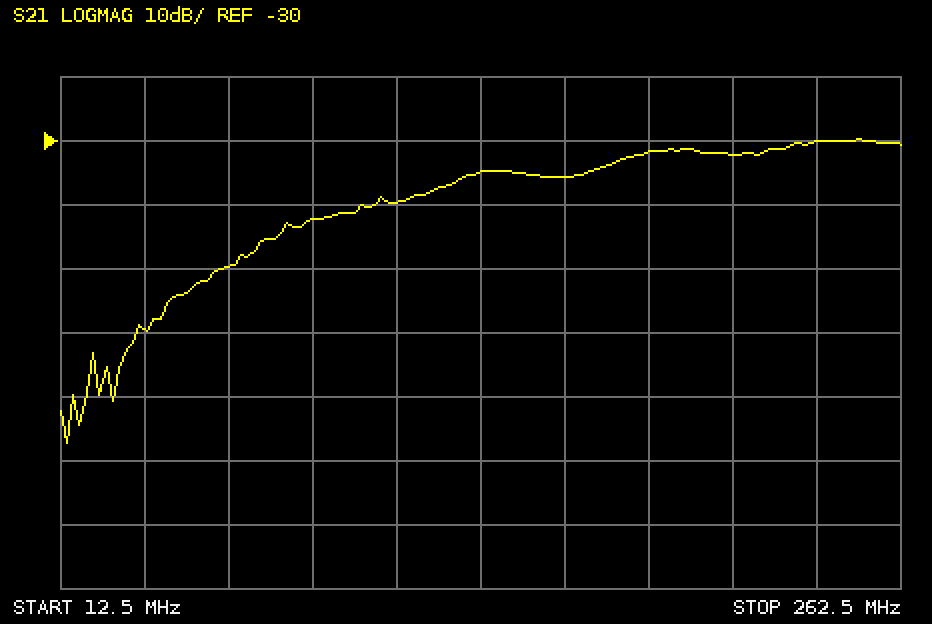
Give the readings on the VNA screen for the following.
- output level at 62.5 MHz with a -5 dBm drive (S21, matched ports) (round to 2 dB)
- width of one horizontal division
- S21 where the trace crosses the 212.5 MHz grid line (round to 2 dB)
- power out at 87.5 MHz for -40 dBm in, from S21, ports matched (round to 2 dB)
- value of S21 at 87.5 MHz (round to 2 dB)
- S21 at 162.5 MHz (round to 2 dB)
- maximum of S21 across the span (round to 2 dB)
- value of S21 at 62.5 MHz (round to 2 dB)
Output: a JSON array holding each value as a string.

["-54 dBm", "25 MHz", "-32 dB", "-82 dBm", "-42 dB", "-36 dB", "-30 dB", "-50 dB"]
